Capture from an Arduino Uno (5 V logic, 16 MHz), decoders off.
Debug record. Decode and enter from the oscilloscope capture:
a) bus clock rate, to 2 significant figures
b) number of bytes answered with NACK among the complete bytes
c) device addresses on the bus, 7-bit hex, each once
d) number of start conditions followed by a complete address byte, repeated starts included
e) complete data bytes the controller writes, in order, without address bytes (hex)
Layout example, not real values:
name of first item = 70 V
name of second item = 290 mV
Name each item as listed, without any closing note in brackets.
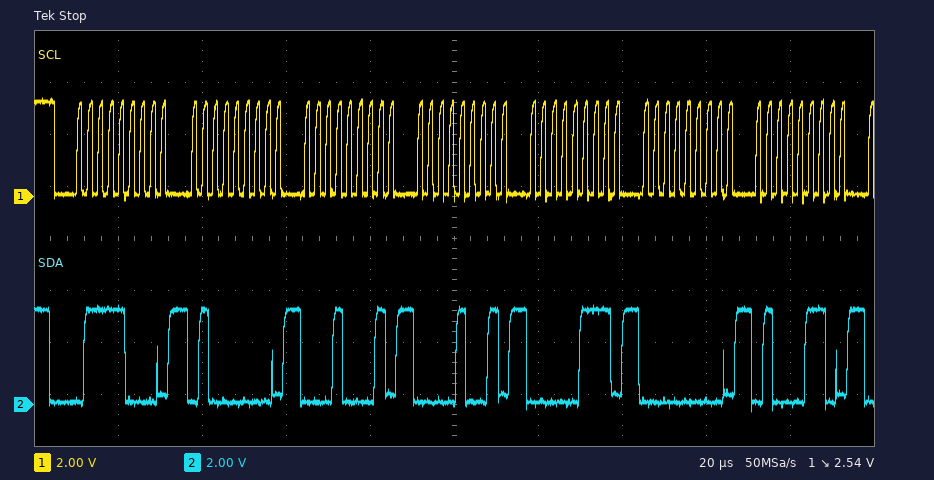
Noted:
bus clock rate, to 2 significant figures = 400 kHz
number of bytes answered with NACK among the complete bytes = 0
device addresses on the bus, 7-bit hex, each once = 0x3C
number of start conditions followed by a complete address byte, repeated starts included = 1
complete data bytes the controller writes, in order, without address bytes = 40 11 09 07 00 46
